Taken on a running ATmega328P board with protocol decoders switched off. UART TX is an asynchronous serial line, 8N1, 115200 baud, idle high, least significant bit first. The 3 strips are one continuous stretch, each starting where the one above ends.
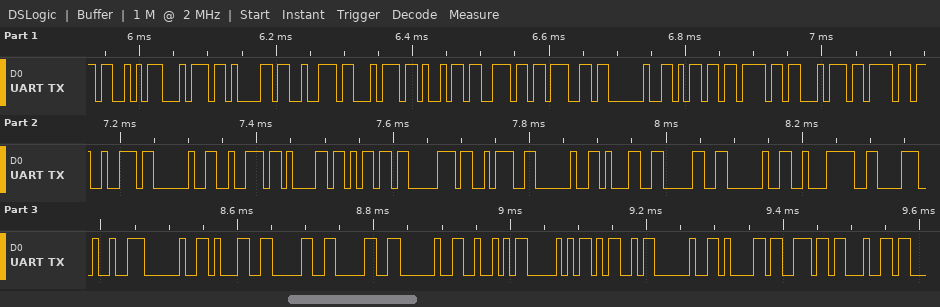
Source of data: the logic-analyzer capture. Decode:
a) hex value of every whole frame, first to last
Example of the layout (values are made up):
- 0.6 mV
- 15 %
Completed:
- 53 74 61 72 74 69 6E 67 20 6D 6F 74 6F 72 20 72 61 6D 70 3A 20 31 30 20 E2 86 92 20 31 30 30 20 52 50 4D 20 61 6E 64
